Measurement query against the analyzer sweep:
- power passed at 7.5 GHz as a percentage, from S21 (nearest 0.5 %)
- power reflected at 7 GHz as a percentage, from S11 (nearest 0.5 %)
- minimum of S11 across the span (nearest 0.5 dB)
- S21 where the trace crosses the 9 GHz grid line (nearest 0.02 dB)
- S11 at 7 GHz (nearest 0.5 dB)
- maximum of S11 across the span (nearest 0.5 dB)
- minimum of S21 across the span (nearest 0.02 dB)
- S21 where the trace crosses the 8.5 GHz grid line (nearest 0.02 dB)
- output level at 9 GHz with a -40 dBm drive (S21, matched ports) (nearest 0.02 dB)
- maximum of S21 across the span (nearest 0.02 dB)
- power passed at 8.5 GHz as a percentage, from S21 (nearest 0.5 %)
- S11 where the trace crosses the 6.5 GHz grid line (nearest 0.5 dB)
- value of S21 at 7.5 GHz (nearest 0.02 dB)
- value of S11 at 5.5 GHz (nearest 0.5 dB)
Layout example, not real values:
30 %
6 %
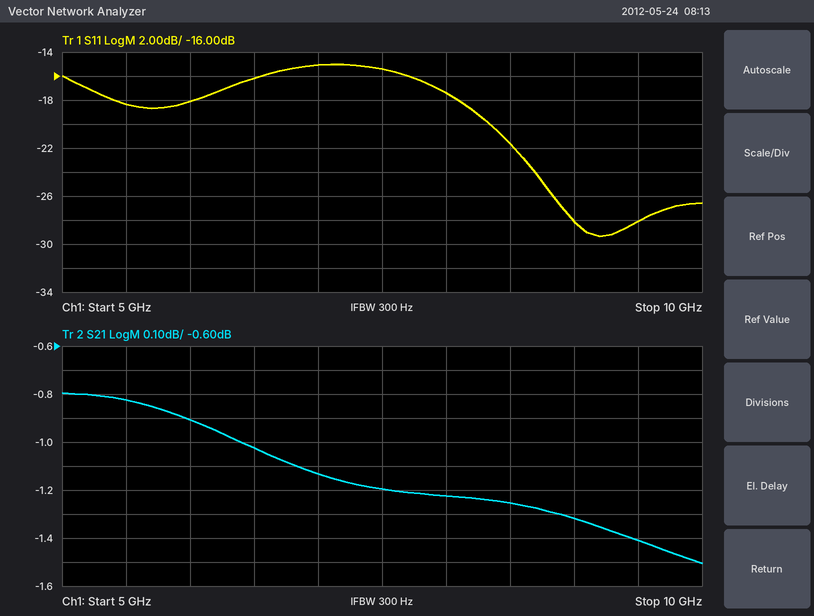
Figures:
76.0 %
3.0 %
-29.5 dB
-1.32 dB
-15.0 dB
-15.0 dB
-1.50 dB
-1.26 dB
-41.32 dBm
-0.80 dB
75.0 %
-16.0 dB
-1.20 dB
-18.5 dB
